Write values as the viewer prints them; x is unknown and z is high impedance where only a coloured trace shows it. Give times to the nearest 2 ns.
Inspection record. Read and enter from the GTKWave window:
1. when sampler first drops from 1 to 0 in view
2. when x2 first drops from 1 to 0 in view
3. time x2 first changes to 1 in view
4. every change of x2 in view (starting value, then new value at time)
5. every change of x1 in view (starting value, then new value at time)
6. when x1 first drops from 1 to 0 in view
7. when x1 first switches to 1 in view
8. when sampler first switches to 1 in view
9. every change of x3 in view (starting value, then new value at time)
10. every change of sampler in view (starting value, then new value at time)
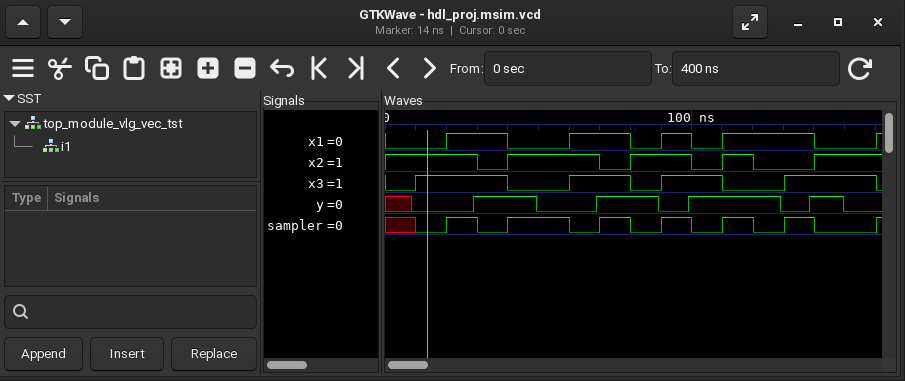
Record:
30 ns
30 ns
40 ns
1, 0 at 30 ns, 1 at 40 ns, 0 at 70 ns, 1 at 80 ns, 0 at 100 ns, 1 at 110 ns, 0 at 120 ns, 1 at 140 ns
0, 1 at 20 ns, 0 at 40 ns, 1 at 60 ns, 0 at 80 ns, 1 at 90 ns, 0 at 100 ns, 1 at 110 ns, 0 at 140 ns, 1 at 160 ns
40 ns
20 ns
20 ns
0, 1 at 10 ns, 0 at 40 ns, 1 at 60 ns, 0 at 80 ns, 1 at 90 ns, 0 at 110 ns, 1 at 130 ns, 0 at 160 ns
x, 0 at 10 ns, 1 at 20 ns, 0 at 30 ns, 1 at 40 ns, 0 at 60 ns, 1 at 70 ns, 0 at 80 ns, 1 at 90 ns, 0 at 100 ns, 1 at 110 ns, 0 at 120 ns, 1 at 130 ns, 0 at 140 ns, 1 at 160 ns
